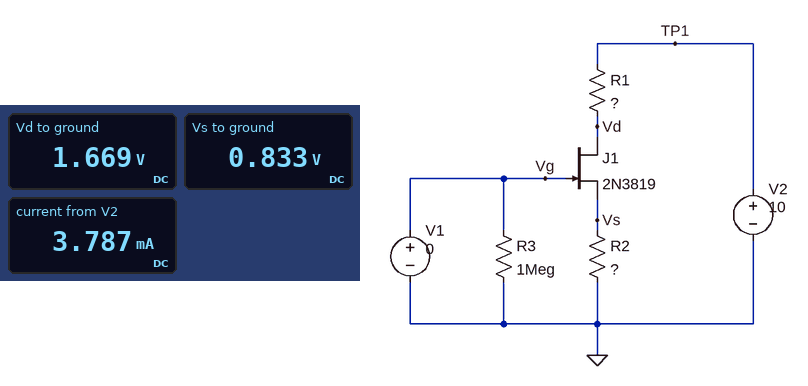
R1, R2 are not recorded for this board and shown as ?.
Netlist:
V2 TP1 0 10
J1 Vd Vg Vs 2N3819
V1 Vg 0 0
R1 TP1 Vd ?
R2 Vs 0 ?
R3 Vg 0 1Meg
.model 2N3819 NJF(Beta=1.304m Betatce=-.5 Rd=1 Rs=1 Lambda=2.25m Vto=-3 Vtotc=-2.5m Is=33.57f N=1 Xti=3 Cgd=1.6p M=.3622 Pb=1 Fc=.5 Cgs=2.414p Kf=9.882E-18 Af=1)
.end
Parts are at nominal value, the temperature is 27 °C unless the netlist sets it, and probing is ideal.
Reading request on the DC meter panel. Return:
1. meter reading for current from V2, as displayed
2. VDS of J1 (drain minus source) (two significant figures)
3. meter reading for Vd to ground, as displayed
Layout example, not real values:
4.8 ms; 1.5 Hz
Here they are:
3.787 mA; 840 mV; 1.669 V
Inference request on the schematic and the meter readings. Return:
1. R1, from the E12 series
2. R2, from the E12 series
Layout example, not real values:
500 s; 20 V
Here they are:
2.2 kΩ; 220 Ω
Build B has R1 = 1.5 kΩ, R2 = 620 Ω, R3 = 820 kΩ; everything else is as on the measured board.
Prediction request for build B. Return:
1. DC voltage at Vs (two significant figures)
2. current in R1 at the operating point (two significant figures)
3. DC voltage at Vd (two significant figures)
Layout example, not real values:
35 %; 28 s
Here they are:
1.6 V; 2.6 mA; 6.1 V
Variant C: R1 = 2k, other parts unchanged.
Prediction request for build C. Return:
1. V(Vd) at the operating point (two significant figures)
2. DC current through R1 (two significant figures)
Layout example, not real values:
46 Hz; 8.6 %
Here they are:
1.9 V; 4.1 mA
